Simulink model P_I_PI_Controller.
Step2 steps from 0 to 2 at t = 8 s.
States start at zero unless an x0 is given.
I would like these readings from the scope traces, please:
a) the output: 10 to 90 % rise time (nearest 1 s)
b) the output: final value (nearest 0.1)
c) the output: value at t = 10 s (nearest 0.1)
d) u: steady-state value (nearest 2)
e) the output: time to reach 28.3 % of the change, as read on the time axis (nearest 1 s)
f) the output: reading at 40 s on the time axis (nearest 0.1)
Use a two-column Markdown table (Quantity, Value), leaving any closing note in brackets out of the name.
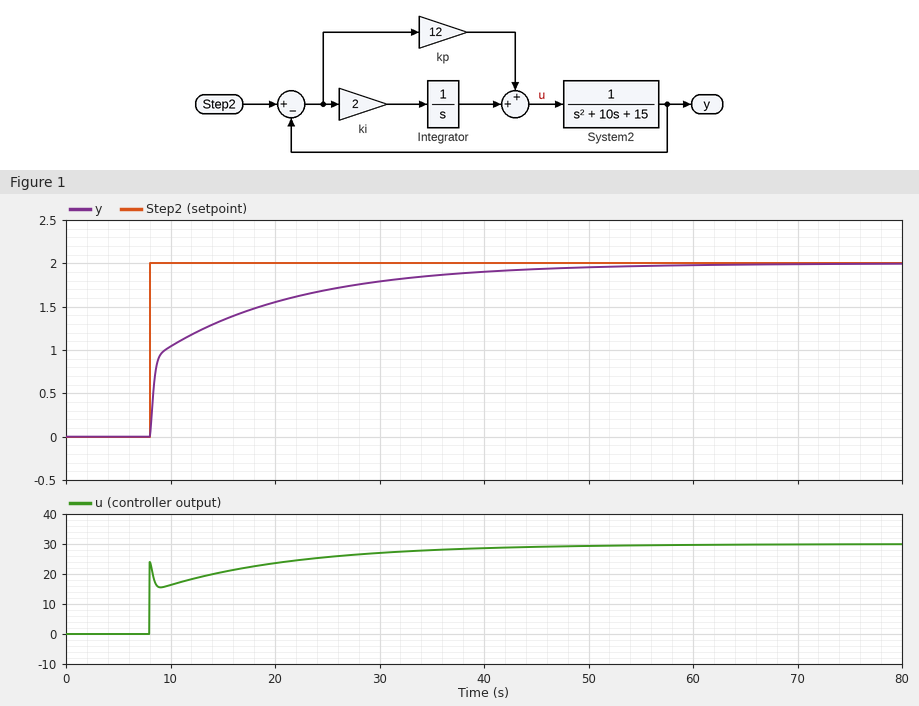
| Quantity | Value |
|---|---|
| the output: 10 to 90 % rise time | 22 s |
| the output: final value | 2.0 |
| the output: value at t = 10 s | 1.0 |
| u: steady-state value | 30 |
| the output: time to reach 28.3 % of the change, as read on the time axis | 8 s |
| the output: reading at 40 s on the time axis | 1.9 |
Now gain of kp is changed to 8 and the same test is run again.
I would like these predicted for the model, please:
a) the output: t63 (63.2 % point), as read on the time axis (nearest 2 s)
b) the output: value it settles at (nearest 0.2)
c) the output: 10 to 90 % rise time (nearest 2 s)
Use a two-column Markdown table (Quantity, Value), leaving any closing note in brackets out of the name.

| Quantity | Value |
|---|---|
| the output: t63 (63.2 % point), as read on the time axis | 14 s |
| the output: value it settles at | 2.0 |
| the output: 10 to 90 % rise time | 20 s |
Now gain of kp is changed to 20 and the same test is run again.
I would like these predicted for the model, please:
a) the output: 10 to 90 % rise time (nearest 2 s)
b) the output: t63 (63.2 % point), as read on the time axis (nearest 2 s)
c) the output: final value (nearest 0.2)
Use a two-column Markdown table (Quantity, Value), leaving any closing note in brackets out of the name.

| Quantity | Value |
|---|---|
| the output: 10 to 90 % rise time | 24 s |
| the output: t63 (63.2 % point), as read on the time axis | 10 s |
| the output: final value | 2.0 |
